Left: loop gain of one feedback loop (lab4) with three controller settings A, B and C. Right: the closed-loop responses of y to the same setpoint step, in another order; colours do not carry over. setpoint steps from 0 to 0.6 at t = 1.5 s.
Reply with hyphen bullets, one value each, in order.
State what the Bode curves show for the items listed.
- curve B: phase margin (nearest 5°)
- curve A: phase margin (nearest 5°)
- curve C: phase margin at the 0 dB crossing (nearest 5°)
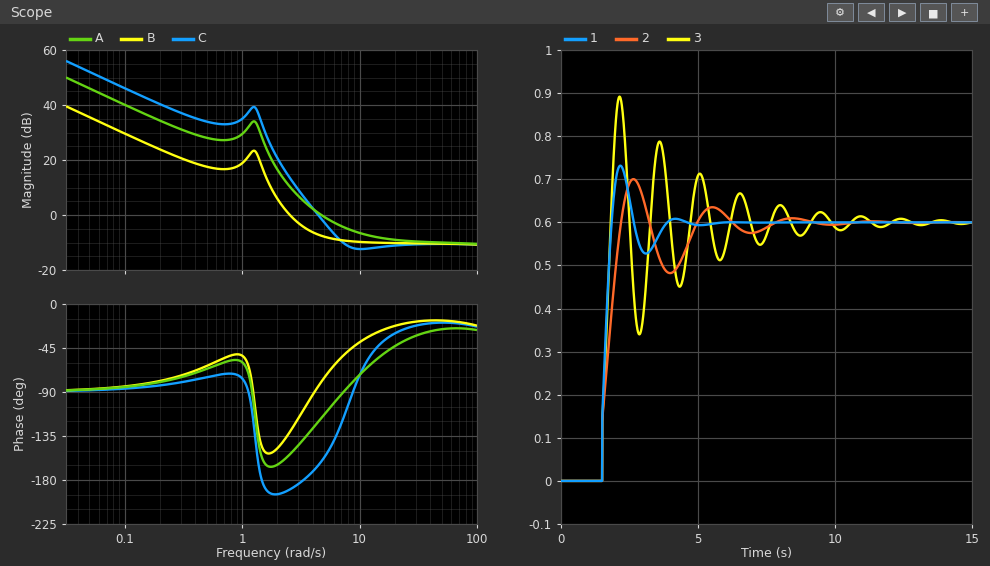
- 50°
- 65°
- 15°
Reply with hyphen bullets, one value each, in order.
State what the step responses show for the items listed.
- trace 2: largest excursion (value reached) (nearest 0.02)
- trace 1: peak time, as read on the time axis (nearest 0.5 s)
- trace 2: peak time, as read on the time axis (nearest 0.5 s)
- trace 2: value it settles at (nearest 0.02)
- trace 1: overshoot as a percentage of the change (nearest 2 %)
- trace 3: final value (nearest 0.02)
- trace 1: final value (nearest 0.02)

- 0.70
- 2.0 s
- 2.5 s
- 0.60
- 22 %
- 0.60
- 0.60
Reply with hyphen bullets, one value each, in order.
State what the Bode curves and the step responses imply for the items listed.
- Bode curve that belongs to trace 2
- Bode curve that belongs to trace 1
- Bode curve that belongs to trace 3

- B
- A
- C
